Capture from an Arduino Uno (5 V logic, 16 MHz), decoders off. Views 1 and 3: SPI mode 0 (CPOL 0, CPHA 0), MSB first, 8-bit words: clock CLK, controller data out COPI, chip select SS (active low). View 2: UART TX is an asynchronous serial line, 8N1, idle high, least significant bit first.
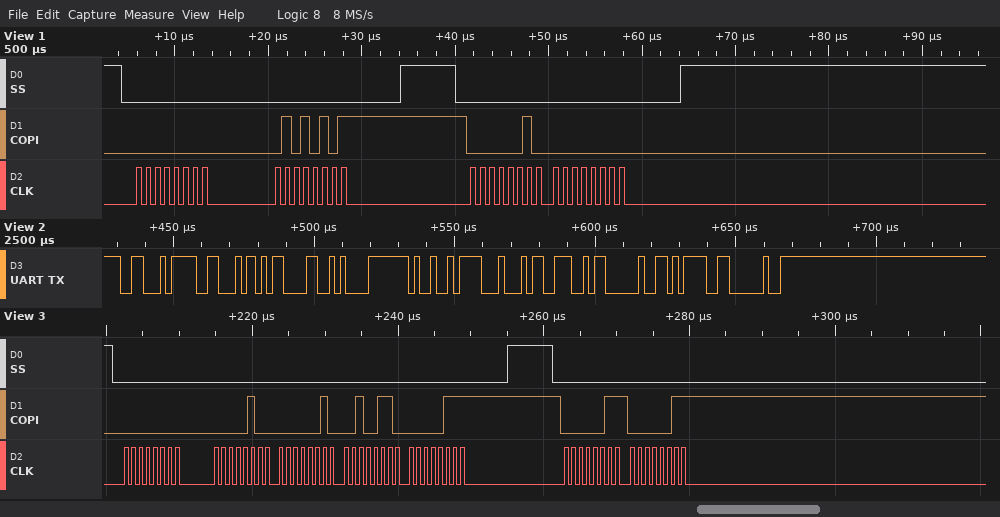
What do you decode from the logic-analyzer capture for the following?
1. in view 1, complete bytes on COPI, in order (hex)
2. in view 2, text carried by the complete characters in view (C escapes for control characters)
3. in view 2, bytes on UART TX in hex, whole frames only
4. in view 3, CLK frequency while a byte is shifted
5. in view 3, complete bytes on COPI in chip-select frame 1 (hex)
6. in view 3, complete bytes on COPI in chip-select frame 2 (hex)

00 55 02 00
"FF\r\nIDN = "
0x46 0x46 0x0D 0x0A 0x49 0x44 0x4E 0x20 0x3D 0x20
1 MHz
00 04 02 26 07
03 03
